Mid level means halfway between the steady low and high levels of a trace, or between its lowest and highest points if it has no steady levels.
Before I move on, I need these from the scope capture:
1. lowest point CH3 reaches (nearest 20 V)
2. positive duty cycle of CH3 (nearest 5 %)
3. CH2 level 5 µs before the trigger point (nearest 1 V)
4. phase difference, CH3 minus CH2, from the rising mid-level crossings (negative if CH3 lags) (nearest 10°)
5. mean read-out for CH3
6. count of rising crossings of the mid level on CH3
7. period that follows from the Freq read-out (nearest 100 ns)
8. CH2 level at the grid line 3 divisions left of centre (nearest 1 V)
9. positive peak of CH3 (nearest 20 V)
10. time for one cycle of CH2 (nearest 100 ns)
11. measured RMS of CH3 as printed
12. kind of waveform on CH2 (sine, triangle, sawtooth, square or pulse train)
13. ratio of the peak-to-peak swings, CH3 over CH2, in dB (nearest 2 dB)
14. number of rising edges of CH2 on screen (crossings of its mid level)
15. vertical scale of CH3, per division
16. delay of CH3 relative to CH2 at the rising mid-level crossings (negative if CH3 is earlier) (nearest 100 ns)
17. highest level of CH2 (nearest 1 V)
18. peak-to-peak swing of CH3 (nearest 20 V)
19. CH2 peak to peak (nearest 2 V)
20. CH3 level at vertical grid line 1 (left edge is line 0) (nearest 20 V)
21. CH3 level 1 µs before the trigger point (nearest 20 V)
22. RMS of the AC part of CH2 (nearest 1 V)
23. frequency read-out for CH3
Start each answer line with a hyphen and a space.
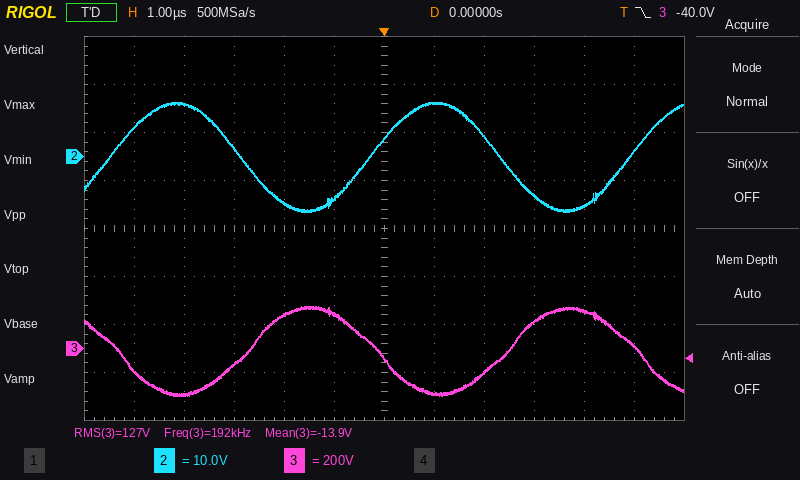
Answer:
- -200 V
- 50 %
- 6 V
- +170°
- -13.9 V
- 2
- 5.2 µs
- 2 V
- 180 V
- 5.2 µs
- 127 V
- sine
- 24 dB
- 3
- 200 V
- -2.4 µs
- 11 V
- 380 V
- 22 V
- -100 V
- 140 V
- 8 V
- 192 kHz
